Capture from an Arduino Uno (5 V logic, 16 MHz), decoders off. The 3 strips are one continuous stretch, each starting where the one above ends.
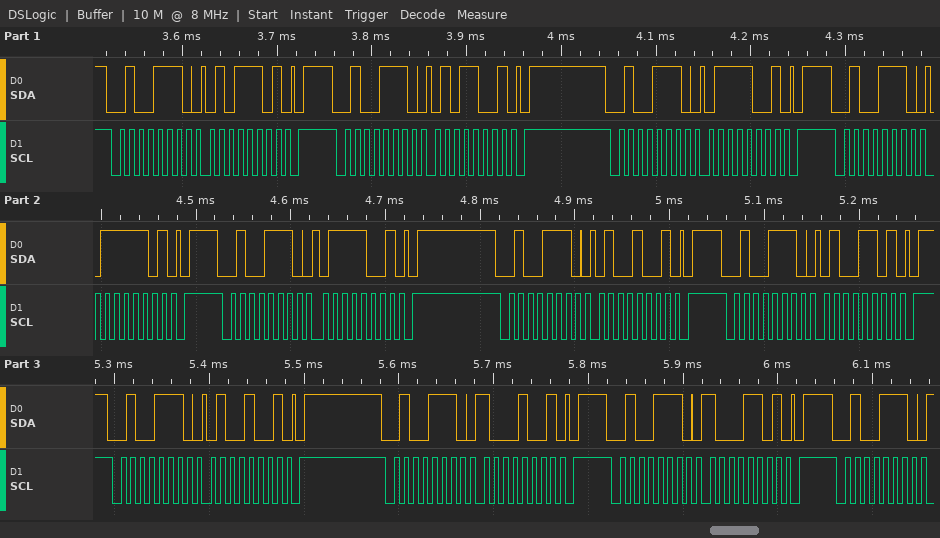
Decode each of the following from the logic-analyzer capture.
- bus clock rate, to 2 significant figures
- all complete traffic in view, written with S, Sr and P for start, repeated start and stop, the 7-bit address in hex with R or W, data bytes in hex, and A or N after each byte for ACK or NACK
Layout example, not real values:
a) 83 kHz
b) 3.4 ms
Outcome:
a) 100 kHz
b) S 27W A 5D A P S 27W A 59 A P S 27W A 79 A P S 27W A 7D A P S 27W A 79 A P S 27W A 49 A P S 27W A 4D A P S 27W A 49 A P S 27W A 89 A P S 27W A 8D A P S 27W A
